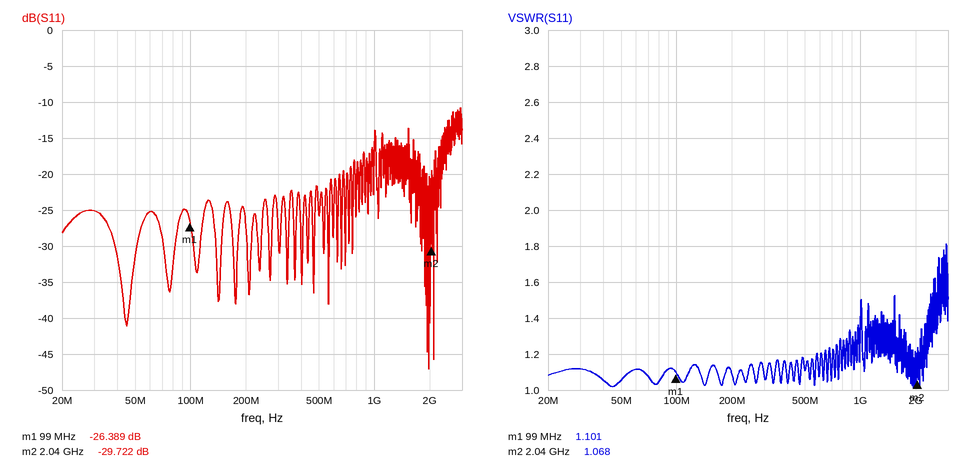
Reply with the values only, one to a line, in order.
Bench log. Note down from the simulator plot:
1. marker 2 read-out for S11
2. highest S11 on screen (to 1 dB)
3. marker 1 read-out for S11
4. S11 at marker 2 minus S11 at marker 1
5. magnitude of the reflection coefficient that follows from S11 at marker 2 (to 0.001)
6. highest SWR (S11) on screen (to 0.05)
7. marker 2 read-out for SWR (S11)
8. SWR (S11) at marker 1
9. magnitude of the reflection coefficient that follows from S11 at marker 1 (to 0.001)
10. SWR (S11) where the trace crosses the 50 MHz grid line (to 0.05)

-29.722 dB
-11 dB
-26.389 dB
-3.333 dB
0.033
1.80
1.068
1.101
0.048
1.05
